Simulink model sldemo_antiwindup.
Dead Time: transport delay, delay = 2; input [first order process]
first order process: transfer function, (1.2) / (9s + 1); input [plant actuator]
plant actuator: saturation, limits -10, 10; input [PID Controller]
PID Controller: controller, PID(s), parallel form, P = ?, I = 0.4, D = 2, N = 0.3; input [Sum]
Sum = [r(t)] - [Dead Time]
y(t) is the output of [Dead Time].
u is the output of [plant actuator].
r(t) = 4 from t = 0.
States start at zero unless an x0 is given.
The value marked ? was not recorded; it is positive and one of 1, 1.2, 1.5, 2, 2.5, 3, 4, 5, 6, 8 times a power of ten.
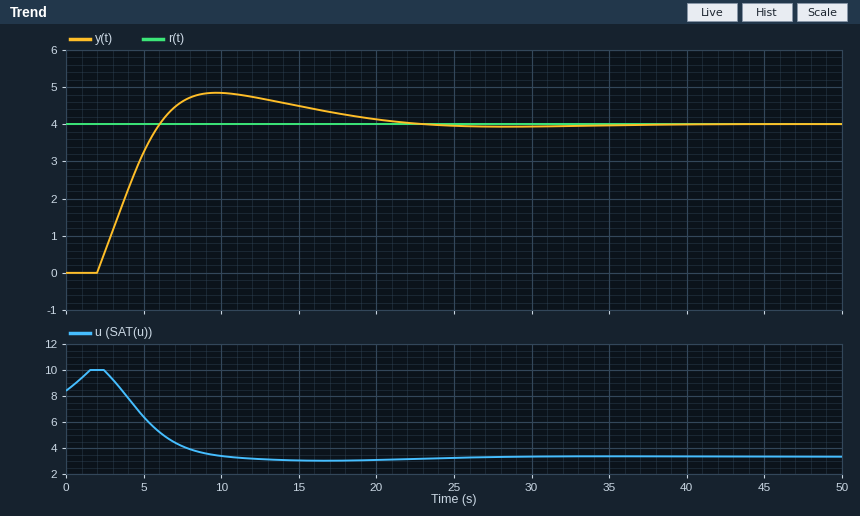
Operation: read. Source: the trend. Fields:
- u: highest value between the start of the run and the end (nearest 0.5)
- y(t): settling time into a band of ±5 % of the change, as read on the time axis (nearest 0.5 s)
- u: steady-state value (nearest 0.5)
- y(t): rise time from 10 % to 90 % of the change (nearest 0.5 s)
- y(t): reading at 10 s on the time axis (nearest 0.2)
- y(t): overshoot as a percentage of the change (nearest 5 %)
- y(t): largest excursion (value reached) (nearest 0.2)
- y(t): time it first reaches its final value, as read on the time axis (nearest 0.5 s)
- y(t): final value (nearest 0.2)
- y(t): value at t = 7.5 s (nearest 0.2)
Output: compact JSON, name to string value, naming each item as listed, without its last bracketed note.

{"u: highest value between the start of the run and the end": "10.0", "y(t): settling time into a band of ±5 % of the change, as read on the time axis": "19.0 s", "u: steady-state value": "3.5", "y(t): rise time from 10 % to 90 % of the change": "3.0 s", "y(t): reading at 10 s on the time axis": "4.8", "y(t): overshoot as a percentage of the change": "20 %", "y(t): largest excursion (value reached)": "4.8", "y(t): time it first reaches its final value, as read on the time axis": "6.0 s", "y(t): final value": "4.0", "y(t): value at t = 7.5 s": "4.6"}
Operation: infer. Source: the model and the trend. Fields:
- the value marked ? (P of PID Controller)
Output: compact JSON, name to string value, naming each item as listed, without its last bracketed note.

{"the value marked ?": "1.5"}
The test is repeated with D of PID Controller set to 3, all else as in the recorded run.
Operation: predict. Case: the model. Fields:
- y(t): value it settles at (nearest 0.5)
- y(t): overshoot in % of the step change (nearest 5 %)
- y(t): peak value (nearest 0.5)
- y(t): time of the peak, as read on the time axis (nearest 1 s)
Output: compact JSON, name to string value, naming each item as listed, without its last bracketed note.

{"y(t): value it settles at": "4.0", "y(t): overshoot in % of the step change": "15 %", "y(t): peak value": "4.5", "y(t): time of the peak, as read on the time axis": "9 s"}
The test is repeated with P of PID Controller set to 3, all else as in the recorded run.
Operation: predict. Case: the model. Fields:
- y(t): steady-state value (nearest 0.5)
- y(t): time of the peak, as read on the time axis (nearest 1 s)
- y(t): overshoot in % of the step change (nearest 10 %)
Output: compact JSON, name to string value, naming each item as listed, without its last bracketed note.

{"y(t): steady-state value": "4.0", "y(t): time of the peak, as read on the time axis": "8 s", "y(t): overshoot in % of the step change": "30 %"}
